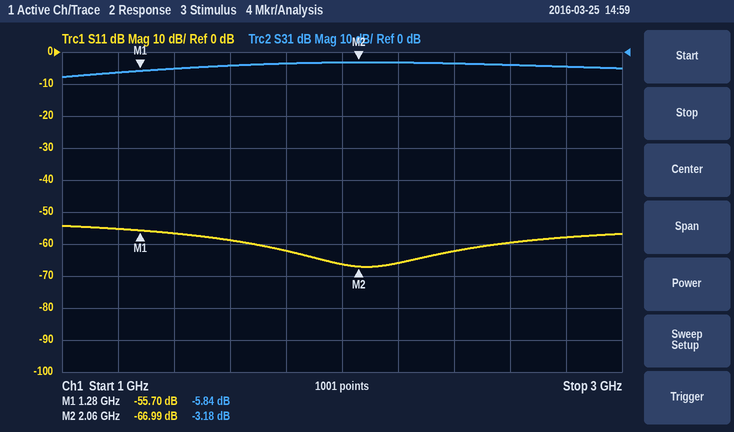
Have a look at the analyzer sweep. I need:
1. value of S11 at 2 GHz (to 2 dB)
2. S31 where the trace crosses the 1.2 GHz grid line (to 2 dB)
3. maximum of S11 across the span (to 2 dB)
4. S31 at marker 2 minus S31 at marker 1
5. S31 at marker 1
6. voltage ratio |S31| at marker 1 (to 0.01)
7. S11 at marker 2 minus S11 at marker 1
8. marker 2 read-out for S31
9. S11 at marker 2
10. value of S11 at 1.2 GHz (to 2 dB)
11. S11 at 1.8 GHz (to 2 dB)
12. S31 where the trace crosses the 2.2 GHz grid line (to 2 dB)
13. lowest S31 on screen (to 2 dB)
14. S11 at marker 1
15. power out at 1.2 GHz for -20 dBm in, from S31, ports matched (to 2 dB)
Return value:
-66 dB
-6 dB
-54 dB
2.66 dB
-5.84 dB
0.51
-11.29 dB
-3.18 dB
-66.99 dB
-56 dB
-62 dB
-4 dB
-8 dB
-55.70 dB
-26 dBm
